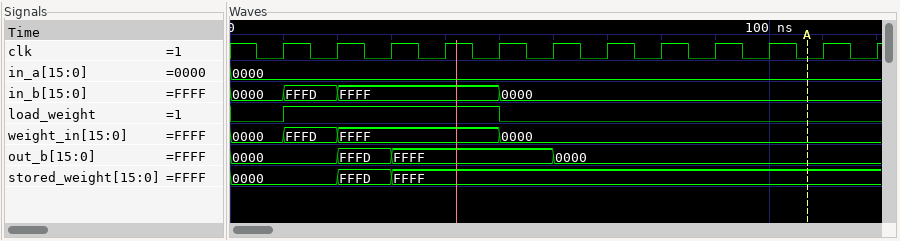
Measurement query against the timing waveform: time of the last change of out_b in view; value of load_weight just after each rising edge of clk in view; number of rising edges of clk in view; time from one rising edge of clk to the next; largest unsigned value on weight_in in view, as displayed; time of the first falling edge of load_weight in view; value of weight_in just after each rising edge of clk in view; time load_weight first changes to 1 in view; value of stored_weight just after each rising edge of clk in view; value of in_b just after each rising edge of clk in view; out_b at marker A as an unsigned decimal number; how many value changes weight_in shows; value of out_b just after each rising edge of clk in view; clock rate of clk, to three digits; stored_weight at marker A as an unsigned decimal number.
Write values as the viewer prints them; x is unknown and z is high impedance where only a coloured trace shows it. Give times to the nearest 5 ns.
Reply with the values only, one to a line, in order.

60 ns
1 1 1 1 0 0 0 0 0 0 0 0
12
10 ns
FFFF
50 ns
FFFD, FFFF, FFFF, FFFF, 0000, 0000, 0000, 0000, 0000, 0000, 0000, 0000
10 ns
0000, FFFD, FFFF, FFFF, FFFF, FFFF, FFFF, FFFF, FFFF, FFFF, FFFF, FFFF
FFFD, FFFF, FFFF, FFFF, 0000, 0000, 0000, 0000, 0000, 0000, 0000, 0000
0
3
0000, FFFD, FFFF, FFFF, FFFF, 0000, 0000, 0000, 0000, 0000, 0000, 0000
100 MHz
65535
